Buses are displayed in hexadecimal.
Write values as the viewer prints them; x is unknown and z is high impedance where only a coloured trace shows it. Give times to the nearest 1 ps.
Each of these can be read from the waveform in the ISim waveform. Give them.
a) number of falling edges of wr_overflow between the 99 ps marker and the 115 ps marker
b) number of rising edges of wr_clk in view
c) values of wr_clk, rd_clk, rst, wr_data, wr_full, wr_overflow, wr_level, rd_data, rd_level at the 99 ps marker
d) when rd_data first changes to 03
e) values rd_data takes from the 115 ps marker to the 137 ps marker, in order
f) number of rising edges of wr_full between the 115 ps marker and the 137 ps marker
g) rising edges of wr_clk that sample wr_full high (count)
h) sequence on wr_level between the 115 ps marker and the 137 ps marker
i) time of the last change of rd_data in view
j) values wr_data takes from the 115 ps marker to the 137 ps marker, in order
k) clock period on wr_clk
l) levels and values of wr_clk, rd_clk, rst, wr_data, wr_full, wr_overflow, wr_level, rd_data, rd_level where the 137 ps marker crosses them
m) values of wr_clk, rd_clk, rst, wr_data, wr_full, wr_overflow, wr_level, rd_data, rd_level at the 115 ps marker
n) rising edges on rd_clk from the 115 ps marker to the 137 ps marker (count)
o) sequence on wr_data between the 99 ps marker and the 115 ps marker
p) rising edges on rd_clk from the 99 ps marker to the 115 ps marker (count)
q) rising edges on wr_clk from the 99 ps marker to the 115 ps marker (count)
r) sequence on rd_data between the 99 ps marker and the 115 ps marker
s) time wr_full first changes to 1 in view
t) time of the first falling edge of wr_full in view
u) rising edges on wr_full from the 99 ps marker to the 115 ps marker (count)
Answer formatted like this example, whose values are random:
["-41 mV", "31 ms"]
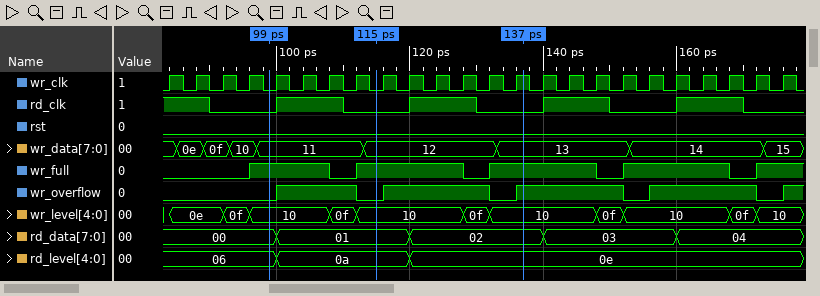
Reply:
["1", "24", "wr_clk=0, rd_clk=0, rst=0, wr_data=11, wr_full=1, wr_overflow=0, wr_level=10, rd_data=00, rd_level=06", "140 ps", "01, 02", "1", "16", "10, 0f, 10", "160 ps", "12, 13", "4 ps", "wr_clk=1, rd_clk=0, rst=0, wr_data=13, wr_full=1, wr_overflow=1, wr_level=10, rd_data=02, rd_level=0e", "wr_clk=0, rd_clk=0, rst=0, wr_data=12, wr_full=1, wr_overflow=0, wr_level=10, rd_data=01, rd_level=0a", "1", "11, 12", "1", "4", "00, 01", "96 ps", "108 ps", "1"]
